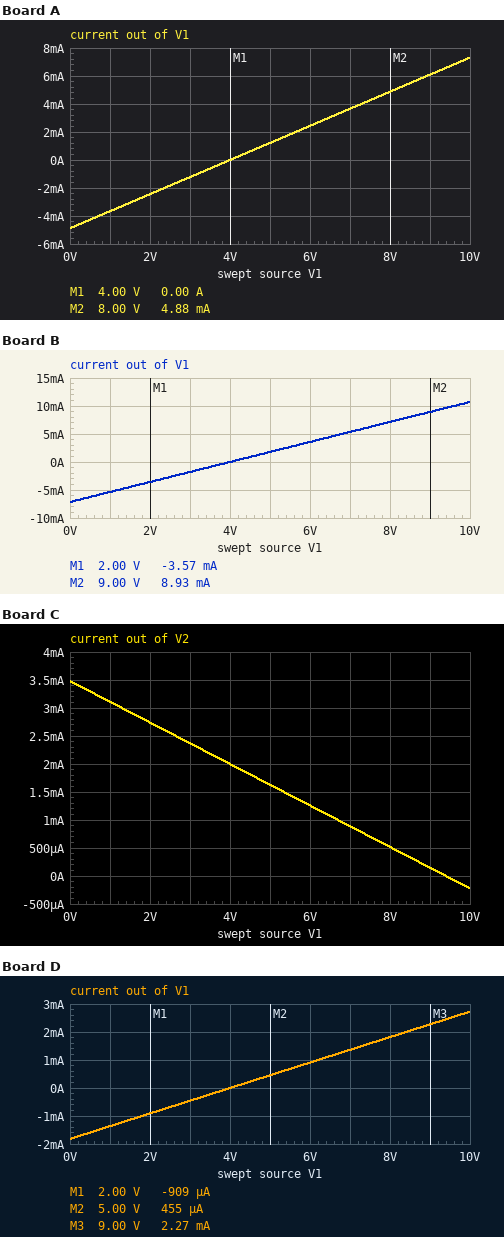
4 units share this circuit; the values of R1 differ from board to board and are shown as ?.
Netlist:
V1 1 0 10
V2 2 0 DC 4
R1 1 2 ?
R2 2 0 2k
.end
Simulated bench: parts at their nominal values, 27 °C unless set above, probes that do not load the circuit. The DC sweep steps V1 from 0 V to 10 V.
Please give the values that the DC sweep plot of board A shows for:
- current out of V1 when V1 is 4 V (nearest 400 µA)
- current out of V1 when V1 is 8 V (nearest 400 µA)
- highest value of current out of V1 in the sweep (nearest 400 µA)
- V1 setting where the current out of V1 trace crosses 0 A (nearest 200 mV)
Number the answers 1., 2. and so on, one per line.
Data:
1. 0 A
2. 4.8 mA
3. 7.2 mA
4. 4.0 V
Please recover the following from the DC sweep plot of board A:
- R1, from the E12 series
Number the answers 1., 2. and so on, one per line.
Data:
1. 820 Ω
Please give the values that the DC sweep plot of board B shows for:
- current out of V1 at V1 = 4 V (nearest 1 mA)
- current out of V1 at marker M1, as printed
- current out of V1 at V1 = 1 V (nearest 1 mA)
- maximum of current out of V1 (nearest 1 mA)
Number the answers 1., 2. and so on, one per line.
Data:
1. 0 A
2. -3.57 mA
3. -5 mA
4. 11 mA
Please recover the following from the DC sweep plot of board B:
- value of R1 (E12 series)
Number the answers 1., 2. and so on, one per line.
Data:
1. 560 Ω
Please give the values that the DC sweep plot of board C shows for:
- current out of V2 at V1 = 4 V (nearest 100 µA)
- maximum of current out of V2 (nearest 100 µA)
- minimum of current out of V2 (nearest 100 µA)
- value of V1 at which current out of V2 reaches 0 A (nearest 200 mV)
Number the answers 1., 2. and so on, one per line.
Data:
1. 2.0 mA
2. 3.5 mA
3. -200 µA
4. 9.4 V
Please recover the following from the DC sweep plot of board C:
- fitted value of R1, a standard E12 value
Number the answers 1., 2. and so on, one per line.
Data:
1. 2.7 kΩ
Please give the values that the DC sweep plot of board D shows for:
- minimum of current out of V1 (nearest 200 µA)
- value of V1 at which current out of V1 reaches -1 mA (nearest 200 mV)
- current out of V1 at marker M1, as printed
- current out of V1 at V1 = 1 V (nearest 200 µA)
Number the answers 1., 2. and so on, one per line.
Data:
1. -1.8 mA
2. 1.8 V
3. -909 µA
4. -1.4 mA
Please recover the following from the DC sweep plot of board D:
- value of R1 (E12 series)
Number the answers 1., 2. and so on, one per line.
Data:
1. 2.2 kΩ
